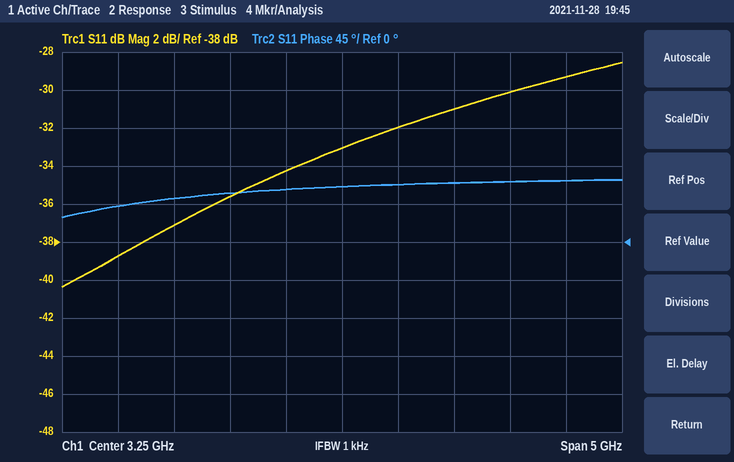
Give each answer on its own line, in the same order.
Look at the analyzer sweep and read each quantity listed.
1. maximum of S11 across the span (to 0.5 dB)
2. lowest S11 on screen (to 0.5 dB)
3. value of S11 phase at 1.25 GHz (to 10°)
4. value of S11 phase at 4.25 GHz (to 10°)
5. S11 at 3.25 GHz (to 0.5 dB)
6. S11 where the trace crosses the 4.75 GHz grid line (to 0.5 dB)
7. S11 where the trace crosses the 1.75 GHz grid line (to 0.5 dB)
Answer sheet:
-28.5 dB
-40.5 dB
40°
70°
-33.0 dB
-30.0 dB
-37.0 dB
